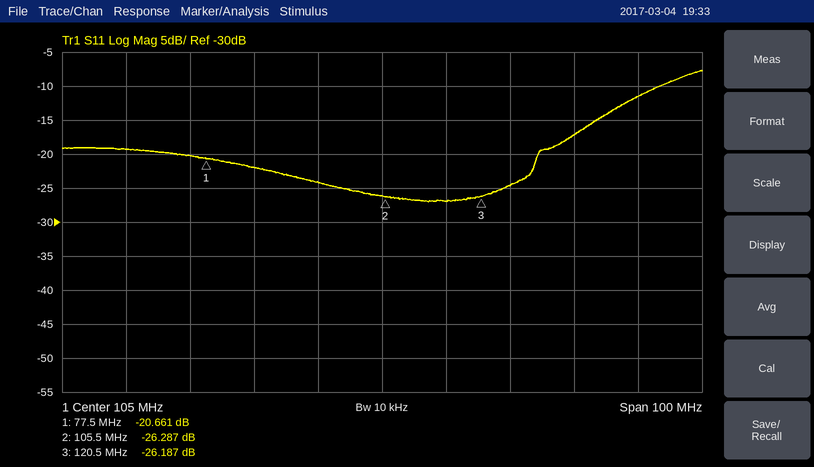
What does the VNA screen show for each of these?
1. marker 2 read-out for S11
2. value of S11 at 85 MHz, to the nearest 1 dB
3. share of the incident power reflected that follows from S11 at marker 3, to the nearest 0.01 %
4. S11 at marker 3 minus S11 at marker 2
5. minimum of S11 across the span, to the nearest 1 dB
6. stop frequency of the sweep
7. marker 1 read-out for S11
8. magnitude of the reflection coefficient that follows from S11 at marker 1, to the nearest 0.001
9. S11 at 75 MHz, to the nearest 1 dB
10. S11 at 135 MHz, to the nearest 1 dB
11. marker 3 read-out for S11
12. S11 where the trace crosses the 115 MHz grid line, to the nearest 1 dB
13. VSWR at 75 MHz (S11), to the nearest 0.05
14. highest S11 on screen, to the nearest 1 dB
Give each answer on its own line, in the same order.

-26.287 dB
-22 dB
0.24 %
0.100 dB
-27 dB
155 MHz
-20.661 dB
0.093
-20 dB
-17 dB
-26.187 dB
-27 dB
1.20
-8 dB
